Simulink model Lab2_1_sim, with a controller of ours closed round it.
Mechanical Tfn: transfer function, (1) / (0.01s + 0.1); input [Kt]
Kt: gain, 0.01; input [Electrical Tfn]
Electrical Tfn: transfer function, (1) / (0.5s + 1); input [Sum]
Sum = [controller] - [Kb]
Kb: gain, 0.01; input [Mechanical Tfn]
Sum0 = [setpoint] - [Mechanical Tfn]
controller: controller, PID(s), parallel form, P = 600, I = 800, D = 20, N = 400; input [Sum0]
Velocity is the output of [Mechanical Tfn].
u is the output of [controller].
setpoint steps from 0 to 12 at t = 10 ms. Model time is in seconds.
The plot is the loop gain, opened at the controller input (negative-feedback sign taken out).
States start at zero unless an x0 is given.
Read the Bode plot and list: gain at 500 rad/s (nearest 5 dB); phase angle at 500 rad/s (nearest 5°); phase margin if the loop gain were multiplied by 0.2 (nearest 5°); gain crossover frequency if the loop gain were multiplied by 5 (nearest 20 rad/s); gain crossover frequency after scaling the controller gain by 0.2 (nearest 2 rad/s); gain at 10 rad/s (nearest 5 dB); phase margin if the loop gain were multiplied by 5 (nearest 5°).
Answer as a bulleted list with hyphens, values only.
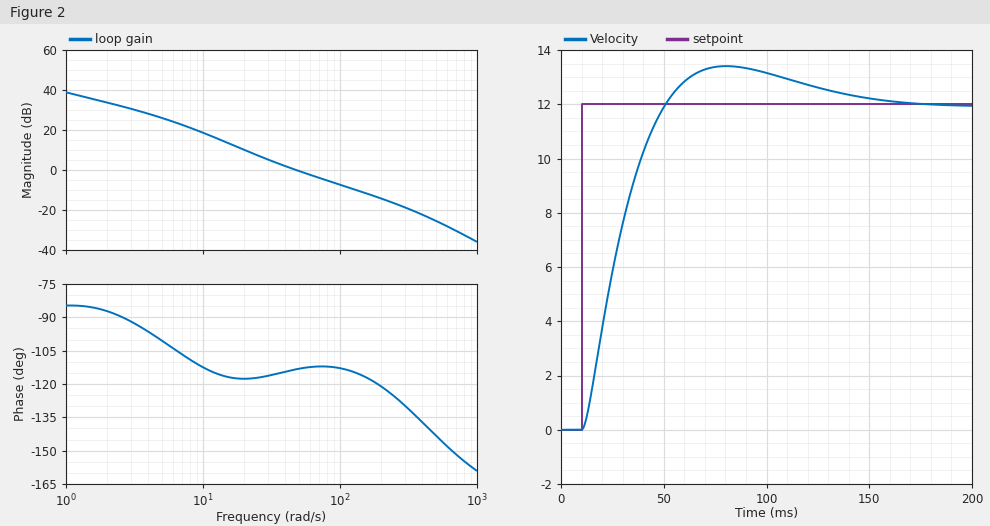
- -25 dB
- -145°
- 65°
- 200 rad/s
- 14 rad/s
- 20 dB
- 60°
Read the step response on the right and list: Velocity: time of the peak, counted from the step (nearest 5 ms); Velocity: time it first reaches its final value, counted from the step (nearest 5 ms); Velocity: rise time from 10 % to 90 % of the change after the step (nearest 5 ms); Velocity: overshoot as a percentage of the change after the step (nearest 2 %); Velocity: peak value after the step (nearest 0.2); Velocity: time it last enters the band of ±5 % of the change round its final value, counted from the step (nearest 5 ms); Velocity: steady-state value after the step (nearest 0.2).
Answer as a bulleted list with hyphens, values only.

- 70 ms
- 40 ms
- 30 ms
- 12 %
- 13.4
- 115 ms
- 12.0
